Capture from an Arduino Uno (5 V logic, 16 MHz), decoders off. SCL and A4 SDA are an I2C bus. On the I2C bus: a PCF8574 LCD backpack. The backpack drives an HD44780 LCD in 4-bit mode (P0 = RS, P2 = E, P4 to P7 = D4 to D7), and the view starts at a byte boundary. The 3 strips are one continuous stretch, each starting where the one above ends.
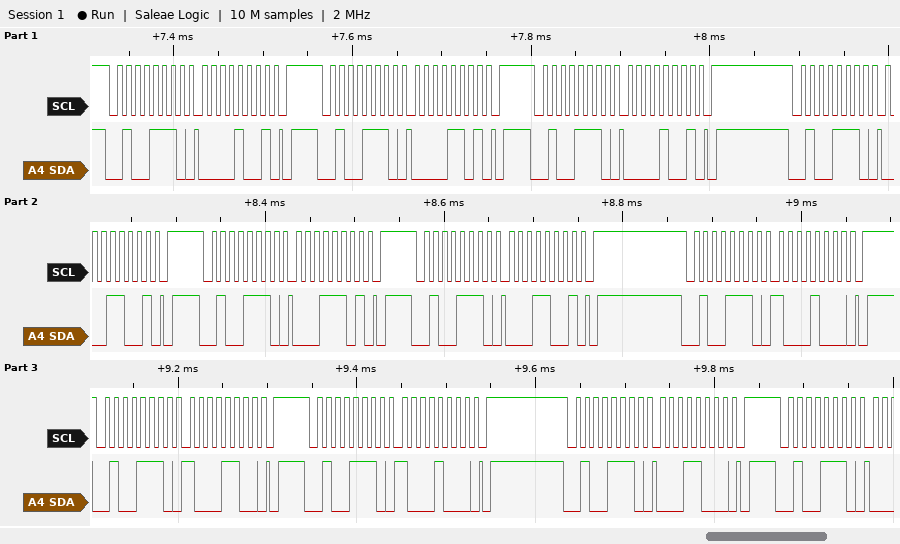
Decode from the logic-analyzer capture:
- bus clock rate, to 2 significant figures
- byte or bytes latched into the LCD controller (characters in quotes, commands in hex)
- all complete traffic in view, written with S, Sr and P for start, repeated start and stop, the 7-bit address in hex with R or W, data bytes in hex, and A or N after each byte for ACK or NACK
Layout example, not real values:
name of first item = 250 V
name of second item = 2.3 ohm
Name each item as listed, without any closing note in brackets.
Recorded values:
bus clock rate, to 2 significant figures = 100 kHz
byte or bytes latched into the LCD controller = data 0x01
all complete traffic in view, written with S, Sr and P for start, repeated start and stop, the 7-bit address in hex with R or W, data bytes in hex, and A or N after each byte for ACK or NACK = S 27W A 09 A P S 27W A 0D A P S 27W A 09 A P S 27W A 19 A P S 27W A 1D A P S 27W A 19 A P S 27W A 88 A P S 27W A 8C A P S 27W A 88 A P S 27W A 18 A P S 27W A
